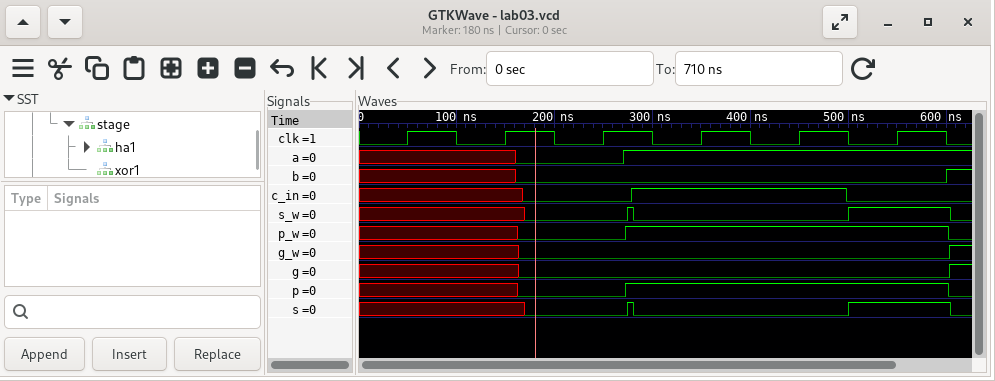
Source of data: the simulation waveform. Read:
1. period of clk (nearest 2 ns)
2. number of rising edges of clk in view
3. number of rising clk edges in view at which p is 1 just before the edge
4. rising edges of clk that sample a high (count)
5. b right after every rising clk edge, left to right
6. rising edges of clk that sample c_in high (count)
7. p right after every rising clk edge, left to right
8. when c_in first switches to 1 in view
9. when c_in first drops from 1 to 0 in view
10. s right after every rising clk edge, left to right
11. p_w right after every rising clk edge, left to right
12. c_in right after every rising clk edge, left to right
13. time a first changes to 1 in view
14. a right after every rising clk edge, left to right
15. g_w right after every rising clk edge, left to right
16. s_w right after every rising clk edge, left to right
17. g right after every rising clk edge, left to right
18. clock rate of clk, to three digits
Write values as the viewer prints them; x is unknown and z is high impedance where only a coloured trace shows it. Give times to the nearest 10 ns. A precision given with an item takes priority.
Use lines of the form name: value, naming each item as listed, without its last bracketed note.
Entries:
period of clk: 100 ns
number of rising edges of clk in view: 6
number of rising clk edges in view at which p is 1 just before the edge: 3
rising edges of clk that sample a high: 3
b right after every rising clk edge, left to right: x x 0 0 0 0
rising edges of clk that sample c_in high: 2
p right after every rising clk edge, left to right: x x 0 1 1 1
when c_in first switches to 1 in view: 280 ns
when c_in first drops from 1 to 0 in view: 500 ns
s right after every rising clk edge, left to right: x x 0 0 0 1
p_w right after every rising clk edge, left to right: x x 0 1 1 1
c_in right after every rising clk edge, left to right: x x 0 1 1 0
time a first changes to 1 in view: 270 ns
a right after every rising clk edge, left to right: x x 0 1 1 1
g_w right after every rising clk edge, left to right: x x 0 0 0 0
s_w right after every rising clk edge, left to right: x x 0 0 0 1
g right after every rising clk edge, left to right: x x 0 0 0 0
clock rate of clk, to three digits: 10.0 MHz
